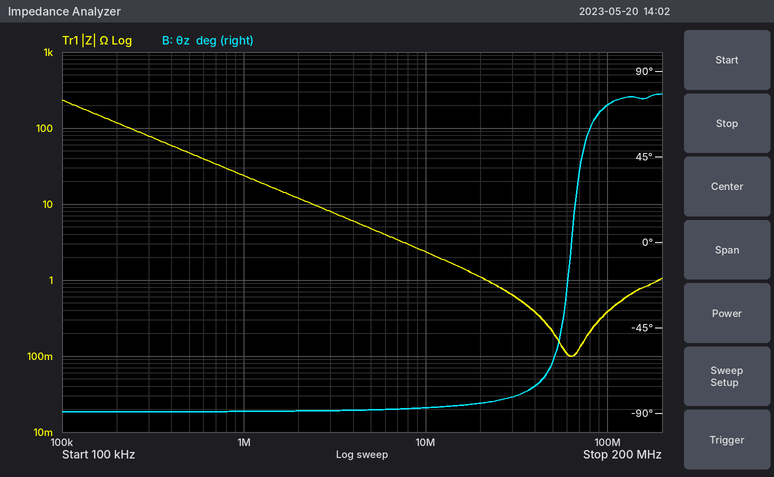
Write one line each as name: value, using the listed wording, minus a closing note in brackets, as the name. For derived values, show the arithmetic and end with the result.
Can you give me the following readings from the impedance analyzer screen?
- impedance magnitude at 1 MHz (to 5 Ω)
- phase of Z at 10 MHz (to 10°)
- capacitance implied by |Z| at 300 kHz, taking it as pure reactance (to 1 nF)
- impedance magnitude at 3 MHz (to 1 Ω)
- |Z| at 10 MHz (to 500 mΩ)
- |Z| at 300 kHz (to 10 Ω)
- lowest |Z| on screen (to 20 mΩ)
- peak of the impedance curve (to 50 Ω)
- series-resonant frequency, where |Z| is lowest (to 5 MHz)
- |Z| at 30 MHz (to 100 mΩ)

impedance magnitude at 1 MHz: 25 Ω
phase of Z at 10 MHz: -90°
capacitance implied by |Z| at 300 kHz, taking it as pure reactance: C = 1/(2π × 300 kHz × 80 Ω) ≈ 7 nF
impedance magnitude at 3 MHz: 8 Ω
|Z| at 10 MHz: 2.5 Ω
|Z| at 300 kHz: 80 Ω
lowest |Z| on screen: 100 mΩ
peak of the impedance curve: 250 Ω
series-resonant frequency, where |Z| is lowest: 65 MHz
|Z| at 30 MHz: 600 mΩ
